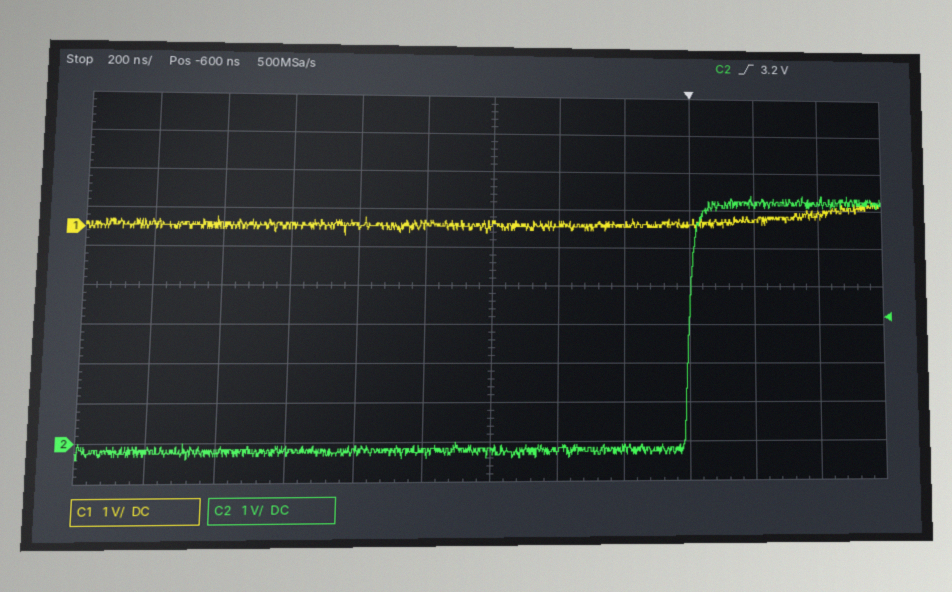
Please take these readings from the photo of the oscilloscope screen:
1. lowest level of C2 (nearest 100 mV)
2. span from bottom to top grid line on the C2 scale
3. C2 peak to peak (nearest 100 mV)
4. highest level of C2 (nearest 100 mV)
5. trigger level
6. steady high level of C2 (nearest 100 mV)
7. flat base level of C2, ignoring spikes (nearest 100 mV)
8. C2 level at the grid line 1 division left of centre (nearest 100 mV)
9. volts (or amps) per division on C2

-400 mV
10 V
6.8 V
6.4 V
3.2 V
6.2 V
-200 mV
-200 mV
1 V
